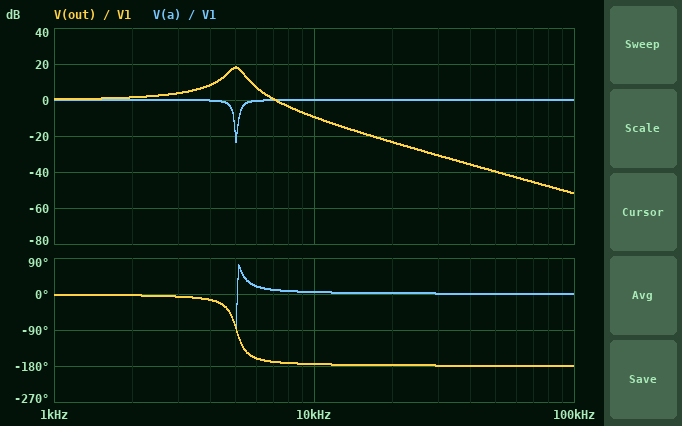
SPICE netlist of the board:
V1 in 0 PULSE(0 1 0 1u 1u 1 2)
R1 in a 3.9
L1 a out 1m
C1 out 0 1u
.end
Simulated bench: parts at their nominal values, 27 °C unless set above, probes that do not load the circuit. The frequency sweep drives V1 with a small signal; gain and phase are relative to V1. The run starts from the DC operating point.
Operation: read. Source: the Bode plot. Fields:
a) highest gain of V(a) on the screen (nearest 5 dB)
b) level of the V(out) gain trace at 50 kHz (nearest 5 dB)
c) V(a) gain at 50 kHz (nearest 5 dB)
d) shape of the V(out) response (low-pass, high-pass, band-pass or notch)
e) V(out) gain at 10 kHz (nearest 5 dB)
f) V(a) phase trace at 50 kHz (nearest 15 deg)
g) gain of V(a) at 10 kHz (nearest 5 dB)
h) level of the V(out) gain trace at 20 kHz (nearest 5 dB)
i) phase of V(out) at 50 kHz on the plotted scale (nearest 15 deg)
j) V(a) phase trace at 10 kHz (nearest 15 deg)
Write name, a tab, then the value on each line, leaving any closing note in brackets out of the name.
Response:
highest gain of V(a) on the screen	0 dB
level of the V(out) gain trace at 50 kHz	-40 dB
V(a) gain at 50 kHz	0 dB
shape of the V(out) response	low-pass
V(out) gain at 10 kHz	-10 dB
V(a) phase trace at 50 kHz	0 deg
gain of V(a) at 10 kHz	0 dB
level of the V(out) gain trace at 20 kHz	-25 dB
phase of V(out) at 50 kHz on the plotted scale	-180 deg
V(a) phase trace at 10 kHz	0 deg
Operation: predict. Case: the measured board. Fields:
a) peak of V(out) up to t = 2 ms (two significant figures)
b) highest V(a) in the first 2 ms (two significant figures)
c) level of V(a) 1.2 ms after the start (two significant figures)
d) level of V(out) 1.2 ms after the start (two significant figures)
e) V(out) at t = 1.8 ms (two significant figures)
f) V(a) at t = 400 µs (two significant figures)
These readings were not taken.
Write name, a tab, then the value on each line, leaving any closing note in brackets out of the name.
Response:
peak of V(out) up to t = 2 ms	1.8 V
highest V(a) in the first 2 ms	1.1 V
level of V(a) 1.2 ms after the start	1.0 V
level of V(out) 1.2 ms after the start	900 mV
V(out) at t = 1.8 ms	970 mV
V(a) at t = 400 µs	1.0 V
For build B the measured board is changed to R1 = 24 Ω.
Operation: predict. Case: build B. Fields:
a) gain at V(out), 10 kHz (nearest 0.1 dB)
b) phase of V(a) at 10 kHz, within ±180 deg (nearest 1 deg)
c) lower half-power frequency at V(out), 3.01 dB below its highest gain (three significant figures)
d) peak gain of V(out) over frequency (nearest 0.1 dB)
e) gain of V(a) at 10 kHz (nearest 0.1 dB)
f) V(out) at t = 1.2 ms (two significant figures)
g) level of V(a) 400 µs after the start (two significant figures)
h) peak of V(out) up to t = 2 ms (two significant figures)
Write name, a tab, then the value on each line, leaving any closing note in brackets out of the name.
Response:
gain at V(out), 10 kHz	-10.4 dB
phase of V(a) at 10 kHz, within ±180 deg	27 deg
lower half-power frequency at V(out), 3.01 dB below its highest gain	499 Hz
peak gain of V(out) over frequency	3.1 dB
gain of V(a) at 10 kHz	-1.0 dB
V(out) at t = 1.2 ms	1.0 V
level of V(a) 400 µs after the start	1.0 V
peak of V(out) up to t = 2 ms	1.3 V
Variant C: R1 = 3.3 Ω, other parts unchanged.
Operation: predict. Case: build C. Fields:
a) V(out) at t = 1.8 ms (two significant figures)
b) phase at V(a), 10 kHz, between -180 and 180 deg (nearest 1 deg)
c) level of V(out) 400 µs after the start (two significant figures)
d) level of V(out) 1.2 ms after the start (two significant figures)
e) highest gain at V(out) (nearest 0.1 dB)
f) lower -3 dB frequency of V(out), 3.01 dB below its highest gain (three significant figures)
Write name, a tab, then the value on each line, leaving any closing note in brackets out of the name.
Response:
V(out) at t = 1.8 ms	950 mV
phase at V(a), 10 kHz, between -180 and 180 deg	4 deg
level of V(out) 400 µs after the start	480 mV
level of V(out) 1.2 ms after the start	860 mV
highest gain at V(out)	19.6 dB
lower -3 dB frequency of V(out), 3.01 dB below its highest gain	4.75 kHz
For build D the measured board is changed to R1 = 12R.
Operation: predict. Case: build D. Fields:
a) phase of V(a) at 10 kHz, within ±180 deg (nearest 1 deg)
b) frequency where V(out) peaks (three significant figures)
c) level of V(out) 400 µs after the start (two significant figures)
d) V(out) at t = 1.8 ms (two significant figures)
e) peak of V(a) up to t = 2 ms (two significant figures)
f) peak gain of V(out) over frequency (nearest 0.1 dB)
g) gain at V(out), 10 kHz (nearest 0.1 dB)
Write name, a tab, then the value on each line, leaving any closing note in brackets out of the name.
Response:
phase of V(a) at 10 kHz, within ±180 deg	14 deg
frequency where V(out) peaks	4.85 kHz
level of V(out) 400 µs after the start	910 mV
V(out) at t = 1.8 ms	1.0 V
peak of V(a) up to t = 2 ms	1.2 V
peak gain of V(out) over frequency	8.6 dB
gain at V(out), 10 kHz	-9.7 dB
